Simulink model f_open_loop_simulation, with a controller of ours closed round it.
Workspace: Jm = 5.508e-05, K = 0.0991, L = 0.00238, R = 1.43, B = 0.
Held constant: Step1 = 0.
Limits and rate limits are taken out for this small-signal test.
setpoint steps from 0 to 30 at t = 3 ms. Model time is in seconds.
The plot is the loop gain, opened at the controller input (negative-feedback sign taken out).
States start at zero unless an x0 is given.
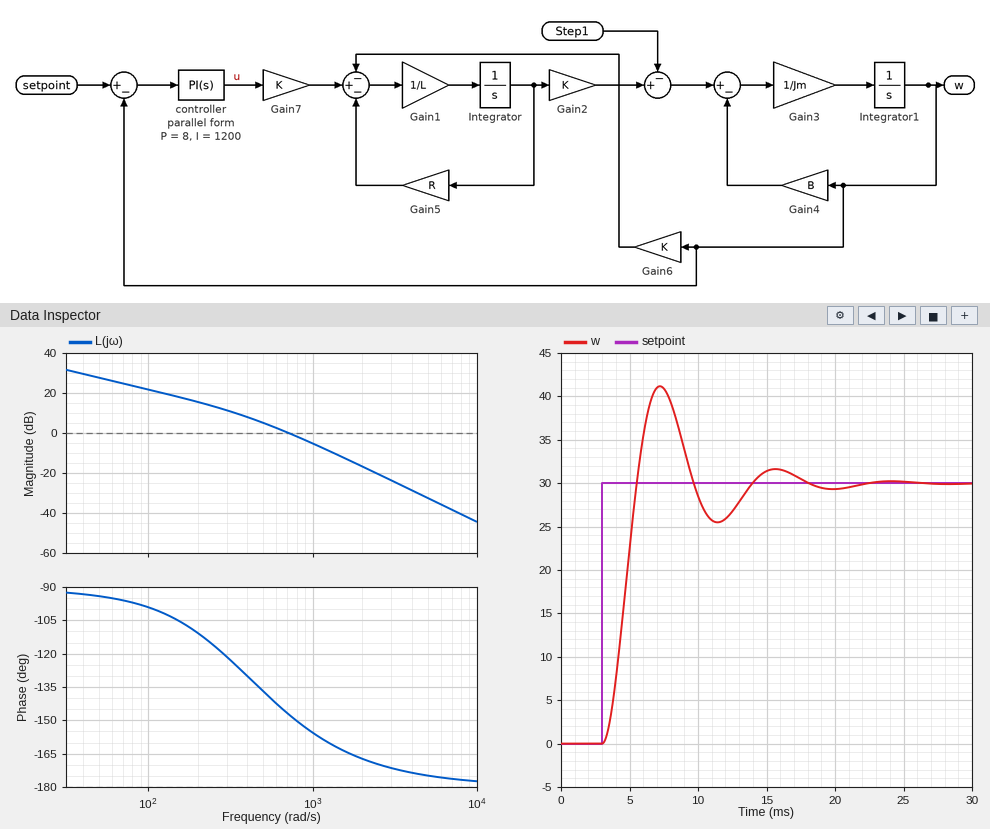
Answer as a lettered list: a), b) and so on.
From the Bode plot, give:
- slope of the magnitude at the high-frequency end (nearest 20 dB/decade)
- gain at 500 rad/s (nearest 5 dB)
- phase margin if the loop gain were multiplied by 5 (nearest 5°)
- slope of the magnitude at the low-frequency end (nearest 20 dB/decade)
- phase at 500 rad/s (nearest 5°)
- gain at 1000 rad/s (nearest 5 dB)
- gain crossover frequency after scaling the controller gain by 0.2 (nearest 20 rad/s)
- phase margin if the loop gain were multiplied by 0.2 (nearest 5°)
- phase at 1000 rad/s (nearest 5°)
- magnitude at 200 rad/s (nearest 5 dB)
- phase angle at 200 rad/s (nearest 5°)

a) -40 dB/decade
b) 5 dB
c) 15°
d) -20 dB/decade
e) -135°
f) -5 dB
g) 240 rad/s
h) 65°
i) -155°
j) 15 dB
k) -110°
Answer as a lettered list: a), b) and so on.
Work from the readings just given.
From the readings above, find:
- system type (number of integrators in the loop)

a) 1
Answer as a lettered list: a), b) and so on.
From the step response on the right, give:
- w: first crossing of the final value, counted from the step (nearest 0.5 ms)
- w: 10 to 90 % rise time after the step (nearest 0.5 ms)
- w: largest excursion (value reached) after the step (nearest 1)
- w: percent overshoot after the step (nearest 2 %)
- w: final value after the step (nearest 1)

a) 2.5 ms
b) 1.5 ms
c) 41
d) 38 %
e) 30
